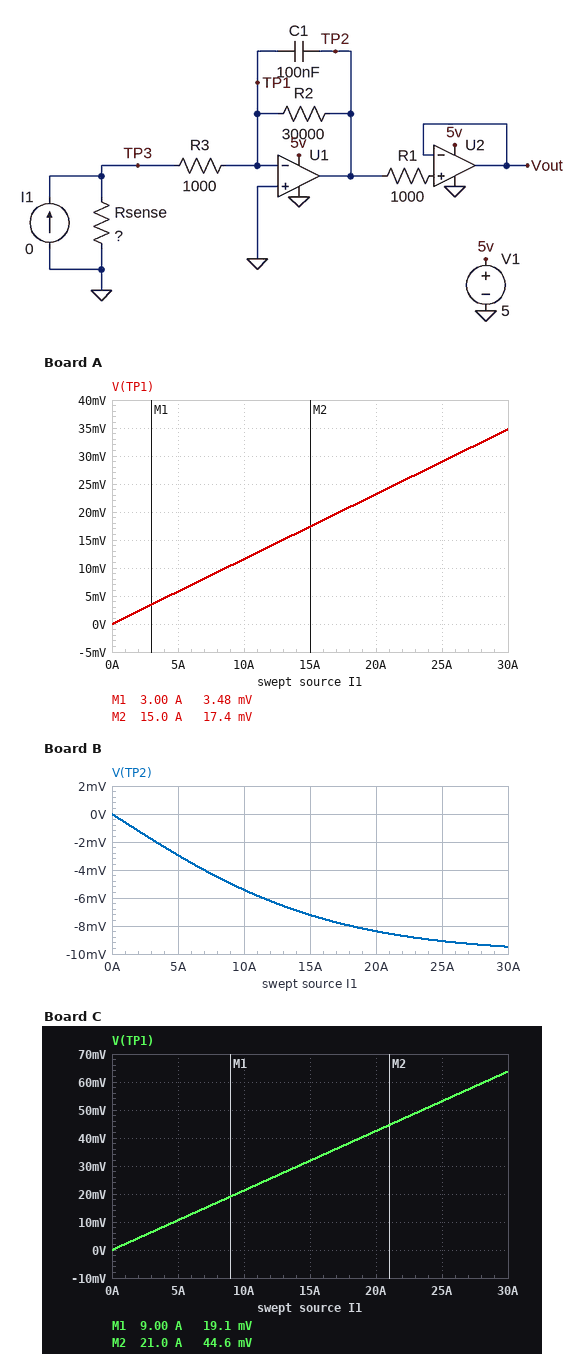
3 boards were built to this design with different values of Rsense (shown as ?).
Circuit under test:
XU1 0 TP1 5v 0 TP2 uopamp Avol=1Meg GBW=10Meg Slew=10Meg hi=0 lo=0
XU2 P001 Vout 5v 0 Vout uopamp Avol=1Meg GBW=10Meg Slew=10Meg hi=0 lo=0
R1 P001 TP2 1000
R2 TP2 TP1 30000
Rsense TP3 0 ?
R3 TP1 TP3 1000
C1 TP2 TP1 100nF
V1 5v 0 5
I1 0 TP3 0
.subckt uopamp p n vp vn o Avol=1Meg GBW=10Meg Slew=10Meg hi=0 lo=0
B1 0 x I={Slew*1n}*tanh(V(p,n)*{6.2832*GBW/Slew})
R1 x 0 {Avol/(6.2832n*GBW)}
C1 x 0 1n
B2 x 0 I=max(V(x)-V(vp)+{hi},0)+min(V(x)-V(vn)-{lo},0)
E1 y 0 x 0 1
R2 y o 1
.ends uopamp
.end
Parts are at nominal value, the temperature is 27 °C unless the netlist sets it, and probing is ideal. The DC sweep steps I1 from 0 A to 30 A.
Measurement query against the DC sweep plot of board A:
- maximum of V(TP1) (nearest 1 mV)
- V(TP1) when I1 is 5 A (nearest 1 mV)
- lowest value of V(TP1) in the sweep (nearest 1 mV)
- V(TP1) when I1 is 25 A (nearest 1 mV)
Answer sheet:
35 mV
6 mV
0 V
29 mV
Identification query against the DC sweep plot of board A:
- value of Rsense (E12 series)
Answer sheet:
1.2 mΩ
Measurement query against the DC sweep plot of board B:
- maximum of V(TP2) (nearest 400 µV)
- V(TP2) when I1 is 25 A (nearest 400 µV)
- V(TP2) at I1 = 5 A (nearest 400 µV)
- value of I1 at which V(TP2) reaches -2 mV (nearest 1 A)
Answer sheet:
0 V
-9.2 mV
-2.8 mV
3 A
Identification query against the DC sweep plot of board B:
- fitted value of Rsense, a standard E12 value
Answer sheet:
0.01 Ω
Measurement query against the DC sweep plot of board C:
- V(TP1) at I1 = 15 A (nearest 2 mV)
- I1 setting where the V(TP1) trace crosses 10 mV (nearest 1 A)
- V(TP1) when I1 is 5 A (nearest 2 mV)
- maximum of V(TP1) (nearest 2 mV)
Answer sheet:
32 mV
5 A
10 mV
64 mV
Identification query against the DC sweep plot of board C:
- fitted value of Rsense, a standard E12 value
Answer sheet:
2.2 mΩ
